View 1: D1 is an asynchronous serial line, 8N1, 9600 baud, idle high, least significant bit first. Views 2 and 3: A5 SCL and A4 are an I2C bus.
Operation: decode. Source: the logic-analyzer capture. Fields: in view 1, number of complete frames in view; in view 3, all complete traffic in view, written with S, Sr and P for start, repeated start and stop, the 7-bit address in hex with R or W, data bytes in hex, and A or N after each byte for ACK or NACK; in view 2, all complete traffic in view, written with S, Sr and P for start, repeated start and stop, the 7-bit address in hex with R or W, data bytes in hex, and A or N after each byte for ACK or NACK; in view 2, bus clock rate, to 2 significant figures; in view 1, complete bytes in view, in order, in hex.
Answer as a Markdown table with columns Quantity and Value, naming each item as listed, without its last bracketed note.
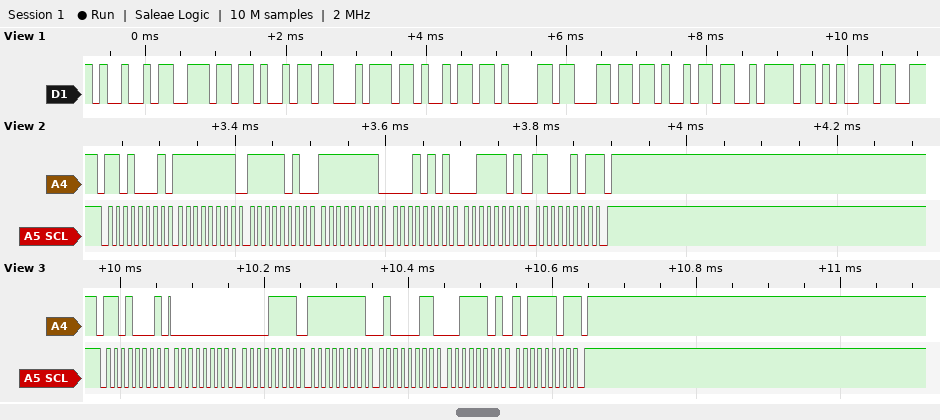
| Quantity | Value |
|---|---|
| in view 1, number of complete frames in view | 10 |
| in view 3, all complete traffic in view, written with S, Sr and P for start, repeated start and stop, the 7-bit address in hex with R or W, data bytes in hex, and A or N after each byte for ACK or NACK | S 68R A 00 A 0F A FF A 43 A 3D A BD N P |
| in view 2, all complete traffic in view, written with S, Sr and P for start, repeated start and stop, the 7-bit address in hex with R or W, data bytes in hex, and A or N after each byte for ACK or NACK | S 68R A FF A FA A FF A 15 A 3D A C5 N P |
| in view 2, bus clock rate, to 2 significant figures | 100 kHz |
| in view 1, complete bytes in view, in order, in hex | 49 6E 69 74 69 61 6C 69 7A 65 |
